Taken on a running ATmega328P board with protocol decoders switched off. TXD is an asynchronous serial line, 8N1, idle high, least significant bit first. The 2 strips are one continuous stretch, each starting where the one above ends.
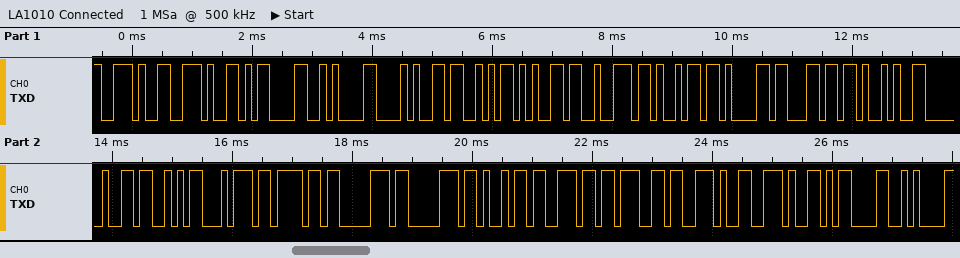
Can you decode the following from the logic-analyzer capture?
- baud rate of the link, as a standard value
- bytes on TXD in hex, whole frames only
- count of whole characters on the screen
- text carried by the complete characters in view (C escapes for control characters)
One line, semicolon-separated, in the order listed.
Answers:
9600 baud; 2E 2E 0D 0A 28 53 65 72 69 61 6C 29 20 53 74 6F 70 70 69 6E 67 2E 2E 0D 0A; 25; "..\r\n(Serial) Stopping..\r\n"
